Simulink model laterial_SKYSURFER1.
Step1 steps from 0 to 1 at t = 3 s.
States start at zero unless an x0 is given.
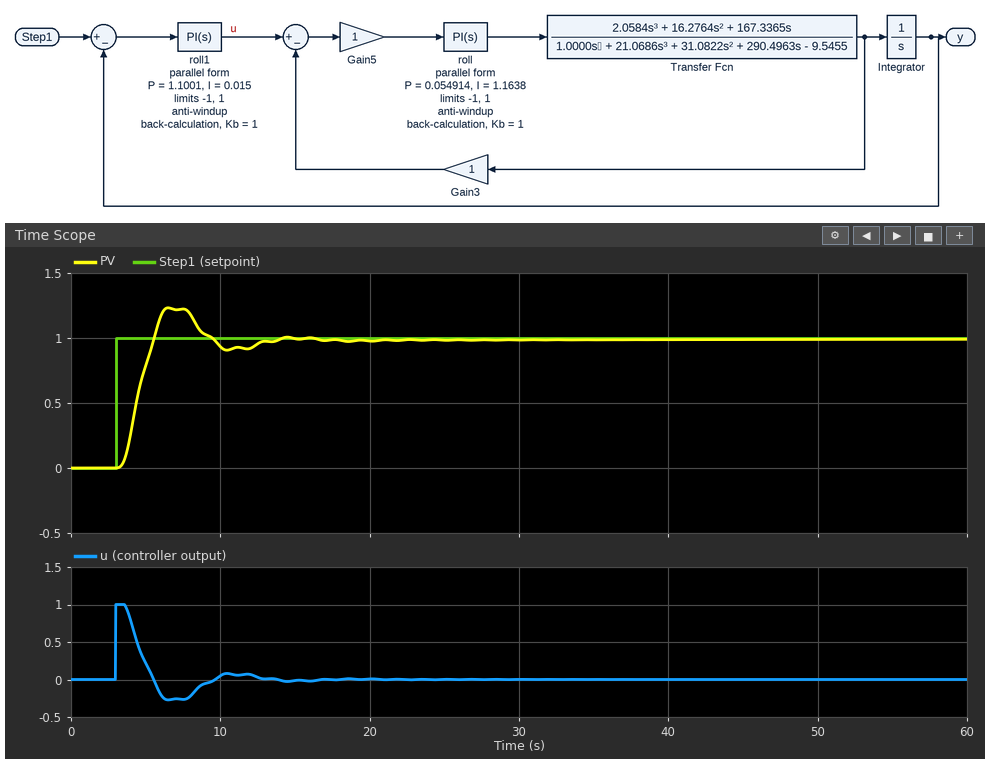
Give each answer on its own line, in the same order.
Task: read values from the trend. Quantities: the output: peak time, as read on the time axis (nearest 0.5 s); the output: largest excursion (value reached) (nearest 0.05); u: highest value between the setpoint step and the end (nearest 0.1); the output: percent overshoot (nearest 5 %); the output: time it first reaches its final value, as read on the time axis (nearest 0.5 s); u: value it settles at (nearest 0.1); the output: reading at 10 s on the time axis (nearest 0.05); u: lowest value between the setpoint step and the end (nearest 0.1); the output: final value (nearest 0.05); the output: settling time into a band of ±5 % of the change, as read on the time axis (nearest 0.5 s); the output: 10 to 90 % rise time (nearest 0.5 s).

6.5 s
1.25
1.0
25 %
5.5 s
0.0
0.95
-0.3
1.00
12.5 s
1.5 s
